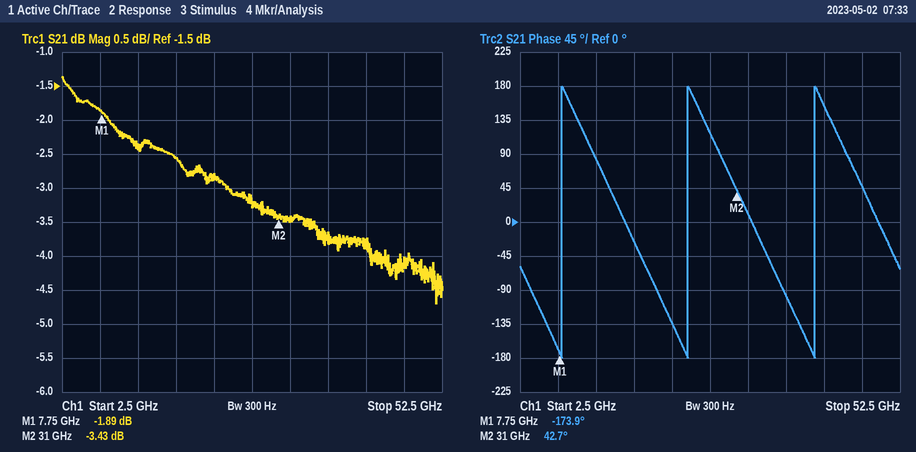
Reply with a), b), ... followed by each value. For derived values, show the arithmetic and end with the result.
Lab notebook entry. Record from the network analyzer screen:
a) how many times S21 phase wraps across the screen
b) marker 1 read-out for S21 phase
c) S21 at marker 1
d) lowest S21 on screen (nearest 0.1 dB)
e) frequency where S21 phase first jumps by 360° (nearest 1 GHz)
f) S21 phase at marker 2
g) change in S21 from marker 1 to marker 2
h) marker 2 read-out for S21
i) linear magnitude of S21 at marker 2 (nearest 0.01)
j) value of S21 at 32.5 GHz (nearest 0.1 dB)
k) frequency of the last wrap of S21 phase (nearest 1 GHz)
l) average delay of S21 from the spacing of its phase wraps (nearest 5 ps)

a) 3
b) -173.9°
c) -1.89 dB
d) -4.7 dB
e) 8 GHz
f) 42.7°
g) -3.43 − (-1.89) = -1.54 dB
h) -3.43 dB
i) 10^(-3.43/20) ≈ 0.67
j) -3.5 dB
k) 41 GHz
l) 2 cycles / (41 GHz − 8 GHz) ≈ 60.6 ps, so 60 ps to the nearest 5 ps
